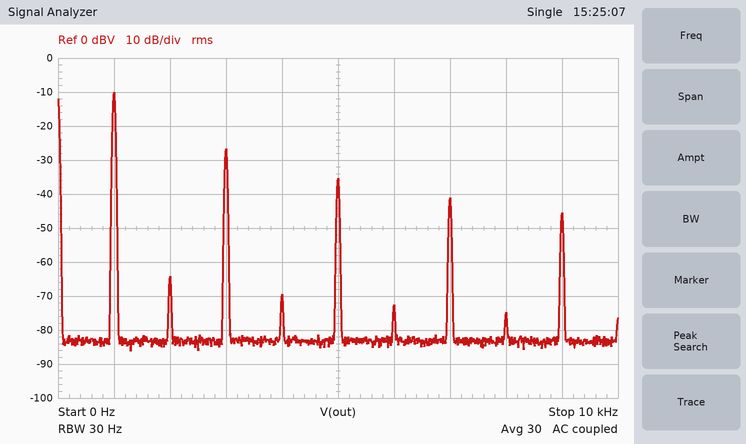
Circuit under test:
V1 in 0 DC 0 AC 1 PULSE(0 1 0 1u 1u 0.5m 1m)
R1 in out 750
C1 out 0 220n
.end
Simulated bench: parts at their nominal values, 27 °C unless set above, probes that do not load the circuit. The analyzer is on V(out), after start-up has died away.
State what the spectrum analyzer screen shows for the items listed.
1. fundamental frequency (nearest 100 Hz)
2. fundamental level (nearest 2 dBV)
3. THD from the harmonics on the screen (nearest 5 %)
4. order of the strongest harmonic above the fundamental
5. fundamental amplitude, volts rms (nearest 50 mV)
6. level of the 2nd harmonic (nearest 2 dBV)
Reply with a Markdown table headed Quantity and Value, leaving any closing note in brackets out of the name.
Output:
| Quantity | Value |
|---|---|
| fundamental frequency | 1.0 kHz |
| fundamental level | -10 dBV |
| THD from the harmonics on the screen | 15 % |
| order of the strongest harmonic above the fundamental | 3 |
| fundamental amplitude, volts rms | 300 mV |
| level of the 2nd harmonic | -64 dBV |
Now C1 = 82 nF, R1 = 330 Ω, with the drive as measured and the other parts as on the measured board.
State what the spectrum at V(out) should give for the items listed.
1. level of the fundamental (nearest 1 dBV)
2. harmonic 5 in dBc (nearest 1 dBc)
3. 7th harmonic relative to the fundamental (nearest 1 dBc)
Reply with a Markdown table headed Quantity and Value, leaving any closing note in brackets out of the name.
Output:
| Quantity | Value |
|---|---|
| level of the fundamental | -7 dBV |
| harmonic 5 in dBc | -16 dBc |
| 7th harmonic relative to the fundamental | -21 dBc |
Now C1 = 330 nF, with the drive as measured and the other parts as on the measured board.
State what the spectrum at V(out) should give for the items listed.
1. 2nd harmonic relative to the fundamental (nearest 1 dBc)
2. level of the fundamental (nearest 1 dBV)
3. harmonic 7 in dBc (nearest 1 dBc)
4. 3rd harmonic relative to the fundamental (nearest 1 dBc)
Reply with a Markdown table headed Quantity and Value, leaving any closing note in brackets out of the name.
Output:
| Quantity | Value |
|---|---|
| 2nd harmonic relative to the fundamental | -55 dBc |
| level of the fundamental | -12 dBV |
| harmonic 7 in dBc | -32 dBc |
| 3rd harmonic relative to the fundamental | -18 dBc |
